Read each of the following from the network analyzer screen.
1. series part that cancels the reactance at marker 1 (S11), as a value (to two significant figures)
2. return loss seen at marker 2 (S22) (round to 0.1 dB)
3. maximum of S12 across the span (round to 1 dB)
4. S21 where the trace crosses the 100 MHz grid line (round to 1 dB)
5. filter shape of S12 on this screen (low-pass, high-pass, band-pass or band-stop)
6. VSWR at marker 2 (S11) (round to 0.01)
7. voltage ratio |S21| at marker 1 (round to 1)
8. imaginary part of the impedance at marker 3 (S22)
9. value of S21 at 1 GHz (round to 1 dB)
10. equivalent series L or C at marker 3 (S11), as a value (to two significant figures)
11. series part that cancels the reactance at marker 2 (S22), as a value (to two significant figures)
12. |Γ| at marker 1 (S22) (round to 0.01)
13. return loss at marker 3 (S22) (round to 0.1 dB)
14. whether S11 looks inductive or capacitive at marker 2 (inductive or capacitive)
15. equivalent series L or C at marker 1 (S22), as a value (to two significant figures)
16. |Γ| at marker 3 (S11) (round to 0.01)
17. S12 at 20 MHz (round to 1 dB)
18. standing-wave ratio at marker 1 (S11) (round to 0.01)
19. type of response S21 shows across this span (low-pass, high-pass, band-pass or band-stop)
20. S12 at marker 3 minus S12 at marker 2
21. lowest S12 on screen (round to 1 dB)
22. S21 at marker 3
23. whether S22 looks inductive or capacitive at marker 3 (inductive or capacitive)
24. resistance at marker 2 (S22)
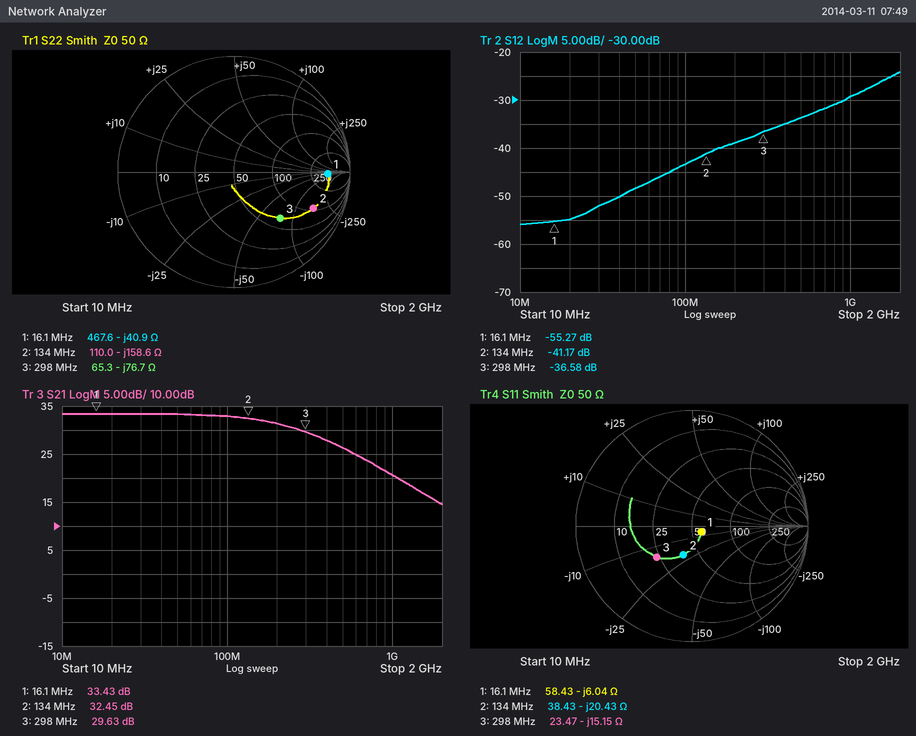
60 nH
2.5 dB
-24 dB
33 dB
high-pass
1.70
47
-76.7 Ω
21 dB
35 pF
190 nH
0.81
5.0 dB
capacitive
240 pF
0.41
-55 dB
1.21
low-pass
4.59 dB
-56 dB
29.63 dB
capacitive
110.0 Ω
